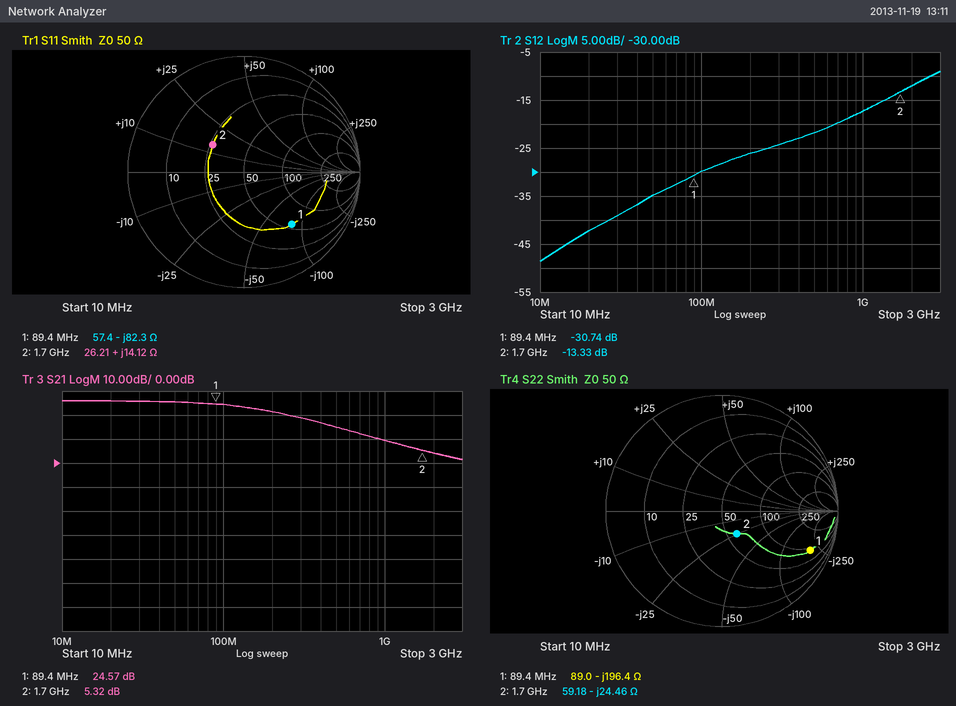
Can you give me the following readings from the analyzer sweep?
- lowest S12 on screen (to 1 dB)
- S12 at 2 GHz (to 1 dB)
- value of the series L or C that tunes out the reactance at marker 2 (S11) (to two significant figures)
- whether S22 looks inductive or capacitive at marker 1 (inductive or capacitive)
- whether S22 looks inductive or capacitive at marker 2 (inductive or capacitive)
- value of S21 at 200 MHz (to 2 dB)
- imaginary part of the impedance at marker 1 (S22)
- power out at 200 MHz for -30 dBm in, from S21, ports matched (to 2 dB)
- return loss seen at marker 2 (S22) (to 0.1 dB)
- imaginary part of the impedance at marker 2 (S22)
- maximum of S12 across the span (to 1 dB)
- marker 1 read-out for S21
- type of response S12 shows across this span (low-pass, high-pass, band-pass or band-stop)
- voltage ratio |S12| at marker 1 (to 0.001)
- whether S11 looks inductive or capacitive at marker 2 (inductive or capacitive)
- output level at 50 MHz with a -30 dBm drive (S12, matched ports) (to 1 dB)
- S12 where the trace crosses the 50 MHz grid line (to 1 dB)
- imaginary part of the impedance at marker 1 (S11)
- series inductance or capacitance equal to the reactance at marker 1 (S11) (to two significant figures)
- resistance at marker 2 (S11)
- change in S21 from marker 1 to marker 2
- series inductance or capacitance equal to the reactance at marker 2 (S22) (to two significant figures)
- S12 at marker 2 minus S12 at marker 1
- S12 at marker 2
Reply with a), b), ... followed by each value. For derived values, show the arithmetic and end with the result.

a) -49 dB
b) -12 dB
c) C = 1/(2π × 1.7 GHz × 14.12 Ω) ≈ 6.6 pF
d) capacitive
e) capacitive
f) 22 dB
g) -196.4 Ω
h) -30 dBm + (22 dB) = -8 dBm
i) 12.6 dB
j) -24.46 Ω
k) -9 dB
l) 24.57 dB
m) high-pass
n) 10^(-30.74/20) ≈ 0.029
o) inductive
p) -30 dBm + (-35 dB) = -65 dBm
q) -35 dB
r) -82.3 Ω
s) C = 1/(2π × 89.4 MHz × 82.3 Ω) ≈ 22 pF
t) 26.21 Ω
u) 5.32 − (24.57) = -19.25 dB
v) C = 1/(2π × 1.7 GHz × 24.46 Ω) ≈ 3.8 pF
w) -13.33 − (-30.74) = 17.41 dB
x) -13.33 dB
